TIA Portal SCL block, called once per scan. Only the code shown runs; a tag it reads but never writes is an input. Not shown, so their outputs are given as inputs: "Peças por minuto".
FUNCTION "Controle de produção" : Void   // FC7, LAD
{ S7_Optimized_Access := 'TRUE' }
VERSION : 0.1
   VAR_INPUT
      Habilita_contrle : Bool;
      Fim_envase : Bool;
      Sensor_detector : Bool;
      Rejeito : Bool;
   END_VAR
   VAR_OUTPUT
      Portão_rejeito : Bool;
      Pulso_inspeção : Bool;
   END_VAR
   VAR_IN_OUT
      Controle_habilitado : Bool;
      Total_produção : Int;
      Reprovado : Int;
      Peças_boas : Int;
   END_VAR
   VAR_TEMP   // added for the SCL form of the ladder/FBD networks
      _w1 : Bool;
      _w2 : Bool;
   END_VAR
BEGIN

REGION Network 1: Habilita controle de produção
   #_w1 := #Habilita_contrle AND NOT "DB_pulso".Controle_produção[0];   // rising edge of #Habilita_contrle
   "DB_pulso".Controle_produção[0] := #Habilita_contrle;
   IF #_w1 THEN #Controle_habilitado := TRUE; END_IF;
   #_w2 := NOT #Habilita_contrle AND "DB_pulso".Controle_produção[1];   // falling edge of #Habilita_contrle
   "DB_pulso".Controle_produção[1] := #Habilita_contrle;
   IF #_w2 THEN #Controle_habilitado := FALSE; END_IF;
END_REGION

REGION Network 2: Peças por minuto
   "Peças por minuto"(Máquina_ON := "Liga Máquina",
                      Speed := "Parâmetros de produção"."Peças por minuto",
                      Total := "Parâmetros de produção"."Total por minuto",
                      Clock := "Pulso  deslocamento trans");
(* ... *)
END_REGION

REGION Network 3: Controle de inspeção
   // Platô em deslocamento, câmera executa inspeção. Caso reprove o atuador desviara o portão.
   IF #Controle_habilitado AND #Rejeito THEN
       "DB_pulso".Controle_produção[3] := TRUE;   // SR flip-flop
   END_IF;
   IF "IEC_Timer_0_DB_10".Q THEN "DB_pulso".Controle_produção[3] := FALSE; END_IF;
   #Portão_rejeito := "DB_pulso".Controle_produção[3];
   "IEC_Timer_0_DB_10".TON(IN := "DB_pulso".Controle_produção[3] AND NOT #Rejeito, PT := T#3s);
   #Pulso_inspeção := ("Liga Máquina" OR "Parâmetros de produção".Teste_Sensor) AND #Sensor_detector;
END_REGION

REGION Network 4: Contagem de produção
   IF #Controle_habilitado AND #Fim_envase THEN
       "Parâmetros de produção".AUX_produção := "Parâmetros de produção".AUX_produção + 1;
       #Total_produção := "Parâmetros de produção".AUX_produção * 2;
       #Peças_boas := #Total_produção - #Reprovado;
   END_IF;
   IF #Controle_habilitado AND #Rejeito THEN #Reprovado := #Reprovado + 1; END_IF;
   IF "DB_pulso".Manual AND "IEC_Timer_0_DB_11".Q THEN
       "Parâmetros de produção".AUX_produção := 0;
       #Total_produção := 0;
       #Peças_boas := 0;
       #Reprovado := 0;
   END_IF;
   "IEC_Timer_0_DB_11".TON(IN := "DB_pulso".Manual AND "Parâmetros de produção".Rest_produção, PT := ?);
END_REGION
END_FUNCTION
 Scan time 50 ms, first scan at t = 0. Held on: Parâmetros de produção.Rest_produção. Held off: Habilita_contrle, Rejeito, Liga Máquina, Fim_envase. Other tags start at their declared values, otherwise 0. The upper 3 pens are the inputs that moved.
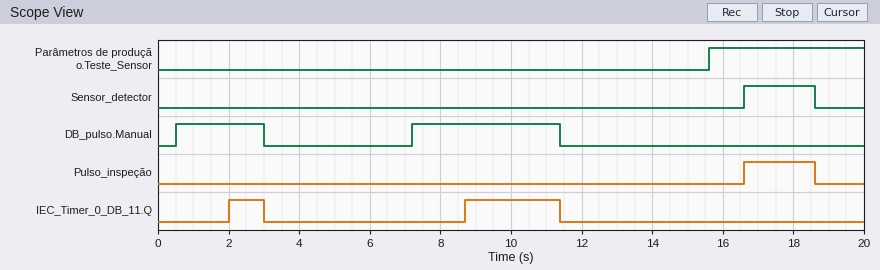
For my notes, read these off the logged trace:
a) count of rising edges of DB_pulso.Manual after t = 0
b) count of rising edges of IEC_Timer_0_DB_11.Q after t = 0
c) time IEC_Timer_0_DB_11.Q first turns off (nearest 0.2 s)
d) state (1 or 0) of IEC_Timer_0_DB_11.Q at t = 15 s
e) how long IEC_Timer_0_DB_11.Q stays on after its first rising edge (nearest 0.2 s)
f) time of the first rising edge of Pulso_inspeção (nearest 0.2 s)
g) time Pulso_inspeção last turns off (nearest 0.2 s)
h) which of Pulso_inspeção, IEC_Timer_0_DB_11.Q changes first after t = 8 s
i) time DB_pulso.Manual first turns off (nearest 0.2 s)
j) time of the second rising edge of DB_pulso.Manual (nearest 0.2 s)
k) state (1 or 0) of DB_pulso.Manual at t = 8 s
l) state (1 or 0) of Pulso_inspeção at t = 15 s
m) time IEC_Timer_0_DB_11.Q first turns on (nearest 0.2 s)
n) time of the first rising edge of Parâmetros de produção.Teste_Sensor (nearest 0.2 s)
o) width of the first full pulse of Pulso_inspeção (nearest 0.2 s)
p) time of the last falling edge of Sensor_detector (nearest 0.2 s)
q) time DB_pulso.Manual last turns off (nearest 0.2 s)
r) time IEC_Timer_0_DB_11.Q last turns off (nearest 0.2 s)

2
2
3.0 s
0
1.0 s
16.6 s
18.6 s
IEC_Timer_0_DB_11.Q
3.0 s
7.2 s
1
0
2.0 s
15.6 s
2.0 s
18.6 s
11.4 s
11.4 s
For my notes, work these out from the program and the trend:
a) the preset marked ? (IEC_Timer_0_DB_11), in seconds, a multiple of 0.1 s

1.5 s
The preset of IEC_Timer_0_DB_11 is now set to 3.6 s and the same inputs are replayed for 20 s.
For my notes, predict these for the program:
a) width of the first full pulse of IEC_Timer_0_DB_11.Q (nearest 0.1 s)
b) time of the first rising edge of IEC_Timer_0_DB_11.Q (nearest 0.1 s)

0.6 s
10.8 s
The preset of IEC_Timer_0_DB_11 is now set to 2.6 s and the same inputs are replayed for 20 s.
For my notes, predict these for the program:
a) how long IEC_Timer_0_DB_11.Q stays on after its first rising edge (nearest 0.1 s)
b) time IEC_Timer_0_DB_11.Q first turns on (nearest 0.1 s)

1.6 s
9.8 s
